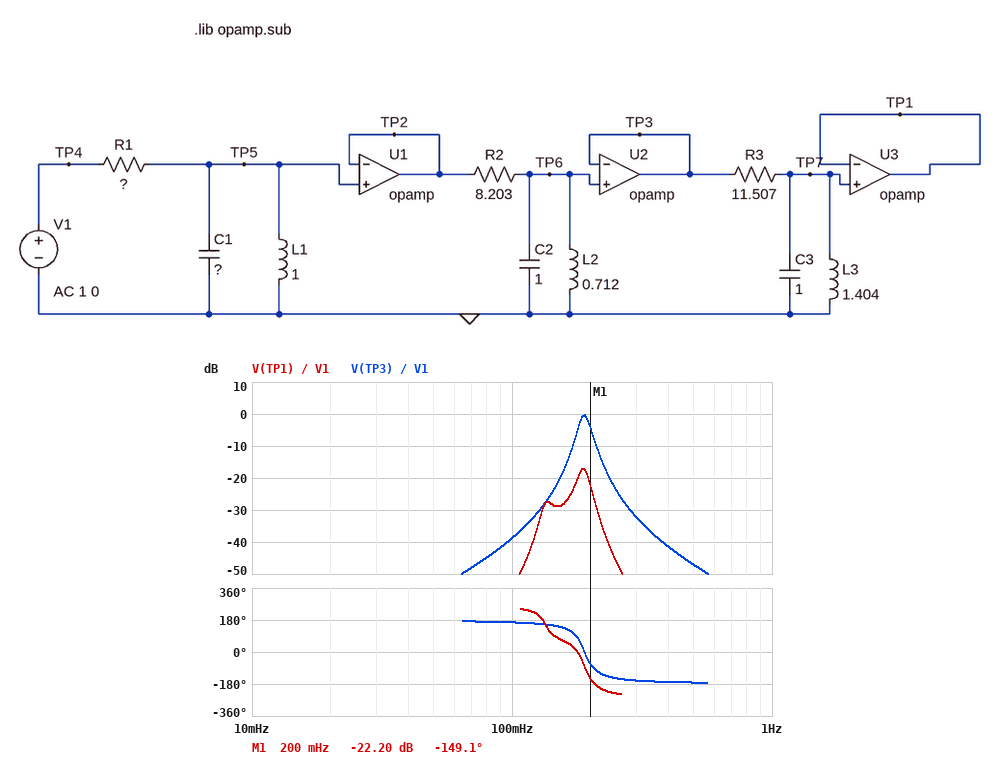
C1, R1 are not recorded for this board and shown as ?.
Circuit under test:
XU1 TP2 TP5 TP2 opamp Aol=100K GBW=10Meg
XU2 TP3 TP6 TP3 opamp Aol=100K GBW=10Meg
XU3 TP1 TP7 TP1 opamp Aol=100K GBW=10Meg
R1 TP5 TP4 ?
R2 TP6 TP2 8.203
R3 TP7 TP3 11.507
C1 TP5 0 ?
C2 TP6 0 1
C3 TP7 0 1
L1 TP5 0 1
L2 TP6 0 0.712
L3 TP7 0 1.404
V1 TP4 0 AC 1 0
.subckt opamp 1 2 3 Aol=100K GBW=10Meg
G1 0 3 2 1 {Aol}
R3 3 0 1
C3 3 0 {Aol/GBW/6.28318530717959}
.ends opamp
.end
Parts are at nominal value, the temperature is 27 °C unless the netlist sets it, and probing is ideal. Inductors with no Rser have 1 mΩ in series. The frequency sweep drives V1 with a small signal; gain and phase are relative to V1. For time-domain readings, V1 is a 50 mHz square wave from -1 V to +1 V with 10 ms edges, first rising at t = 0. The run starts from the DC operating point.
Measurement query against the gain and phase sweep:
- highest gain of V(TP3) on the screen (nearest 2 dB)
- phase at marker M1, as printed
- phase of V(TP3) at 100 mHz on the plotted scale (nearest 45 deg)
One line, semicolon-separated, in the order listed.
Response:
0 dB; -149.1 deg; 180 deg
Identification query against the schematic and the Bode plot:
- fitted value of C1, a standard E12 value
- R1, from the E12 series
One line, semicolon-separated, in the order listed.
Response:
680 mF; 5.6 Ω
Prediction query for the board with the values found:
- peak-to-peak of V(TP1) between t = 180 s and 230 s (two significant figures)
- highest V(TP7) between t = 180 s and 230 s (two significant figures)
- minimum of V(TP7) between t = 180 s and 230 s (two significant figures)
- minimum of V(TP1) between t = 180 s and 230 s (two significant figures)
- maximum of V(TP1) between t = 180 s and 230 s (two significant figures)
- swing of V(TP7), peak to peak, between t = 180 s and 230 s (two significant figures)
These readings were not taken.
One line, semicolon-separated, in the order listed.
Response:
32 mV; 16 mV; -16 mV; -16 mV; 16 mV; 32 mV
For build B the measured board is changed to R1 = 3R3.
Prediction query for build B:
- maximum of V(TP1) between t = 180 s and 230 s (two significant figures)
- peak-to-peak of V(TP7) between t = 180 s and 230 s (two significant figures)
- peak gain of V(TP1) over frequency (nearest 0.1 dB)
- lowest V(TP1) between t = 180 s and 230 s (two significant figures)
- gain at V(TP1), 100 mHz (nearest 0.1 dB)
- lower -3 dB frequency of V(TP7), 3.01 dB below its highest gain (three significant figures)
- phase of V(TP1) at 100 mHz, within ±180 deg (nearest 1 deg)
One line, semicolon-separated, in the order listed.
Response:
24 mV; 49 mV; -16.8 dB; -24 mV; -49.8 dB; 177 mHz; -119 deg
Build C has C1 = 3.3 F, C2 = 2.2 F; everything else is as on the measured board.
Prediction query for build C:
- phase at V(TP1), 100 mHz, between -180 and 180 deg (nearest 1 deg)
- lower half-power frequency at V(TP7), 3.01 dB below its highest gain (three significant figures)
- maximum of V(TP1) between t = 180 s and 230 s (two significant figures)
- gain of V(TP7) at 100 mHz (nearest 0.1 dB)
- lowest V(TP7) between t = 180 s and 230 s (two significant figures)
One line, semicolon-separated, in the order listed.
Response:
92 deg; 124 mHz; 3.3 mV; -41.6 dB; -3.3 mV
